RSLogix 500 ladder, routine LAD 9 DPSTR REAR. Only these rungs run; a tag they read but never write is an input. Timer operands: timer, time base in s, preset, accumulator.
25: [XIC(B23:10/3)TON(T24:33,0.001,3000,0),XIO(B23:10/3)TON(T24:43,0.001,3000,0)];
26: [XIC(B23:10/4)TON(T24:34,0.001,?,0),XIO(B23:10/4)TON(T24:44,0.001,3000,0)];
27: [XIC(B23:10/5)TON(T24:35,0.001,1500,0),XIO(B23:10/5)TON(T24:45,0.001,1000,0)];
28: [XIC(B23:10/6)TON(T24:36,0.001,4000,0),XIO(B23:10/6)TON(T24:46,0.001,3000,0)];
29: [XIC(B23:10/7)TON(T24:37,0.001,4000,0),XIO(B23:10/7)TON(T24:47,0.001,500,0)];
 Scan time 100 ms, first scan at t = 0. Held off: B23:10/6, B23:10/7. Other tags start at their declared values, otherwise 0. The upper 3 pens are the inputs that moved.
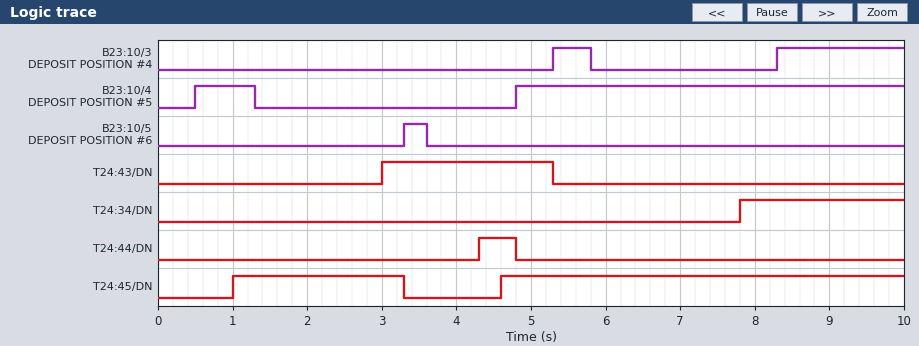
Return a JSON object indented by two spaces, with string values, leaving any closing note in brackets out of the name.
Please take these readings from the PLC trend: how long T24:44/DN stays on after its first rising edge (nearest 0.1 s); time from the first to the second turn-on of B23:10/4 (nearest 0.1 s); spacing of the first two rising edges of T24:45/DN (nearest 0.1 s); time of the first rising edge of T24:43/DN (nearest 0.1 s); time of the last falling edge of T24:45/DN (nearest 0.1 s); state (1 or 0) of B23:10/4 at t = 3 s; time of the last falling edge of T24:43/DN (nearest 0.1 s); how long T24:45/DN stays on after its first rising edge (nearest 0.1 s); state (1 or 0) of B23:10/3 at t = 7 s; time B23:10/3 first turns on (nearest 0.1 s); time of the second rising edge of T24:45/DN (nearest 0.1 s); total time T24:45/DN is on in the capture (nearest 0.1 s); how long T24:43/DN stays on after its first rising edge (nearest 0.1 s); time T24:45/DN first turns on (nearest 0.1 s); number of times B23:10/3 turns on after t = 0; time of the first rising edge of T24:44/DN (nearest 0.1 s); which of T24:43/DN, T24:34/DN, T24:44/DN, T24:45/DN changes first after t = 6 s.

{
  "how long T24:44/DN stays on after its first rising edge": "0.5 s",
  "time from the first to the second turn-on of B23:10/4": "4.3 s",
  "spacing of the first two rising edges of T24:45/DN": "3.6 s",
  "time of the first rising edge of T24:43/DN": "3.0 s",
  "time of the last falling edge of T24:45/DN": "3.3 s",
  "state (1 or 0) of B23:10/4 at t = 3 s": "0",
  "time of the last falling edge of T24:43/DN": "5.3 s",
  "how long T24:45/DN stays on after its first rising edge": "2.3 s",
  "state (1 or 0) of B23:10/3 at t = 7 s": "0",
  "time B23:10/3 first turns on": "5.3 s",
  "time of the second rising edge of T24:45/DN": "4.6 s",
  "total time T24:45/DN is on in the capture": "7.7 s",
  "how long T24:43/DN stays on after its first rising edge": "2.3 s",
  "time T24:45/DN first turns on": "1.0 s",
  "number of times B23:10/3 turns on after t = 0": "2",
  "time of the first rising edge of T24:44/DN": "4.3 s",
  "which of T24:43/DN, T24:34/DN, T24:44/DN, T24:45/DN changes first after t = 6 s": "T24:34/DN"
}
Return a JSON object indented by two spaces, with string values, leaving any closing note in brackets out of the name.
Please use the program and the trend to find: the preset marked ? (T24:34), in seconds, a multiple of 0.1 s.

{
  "the preset marked ? (T24:34), in seconds, a multiple of 0.1 s": "3.0 s"
}
